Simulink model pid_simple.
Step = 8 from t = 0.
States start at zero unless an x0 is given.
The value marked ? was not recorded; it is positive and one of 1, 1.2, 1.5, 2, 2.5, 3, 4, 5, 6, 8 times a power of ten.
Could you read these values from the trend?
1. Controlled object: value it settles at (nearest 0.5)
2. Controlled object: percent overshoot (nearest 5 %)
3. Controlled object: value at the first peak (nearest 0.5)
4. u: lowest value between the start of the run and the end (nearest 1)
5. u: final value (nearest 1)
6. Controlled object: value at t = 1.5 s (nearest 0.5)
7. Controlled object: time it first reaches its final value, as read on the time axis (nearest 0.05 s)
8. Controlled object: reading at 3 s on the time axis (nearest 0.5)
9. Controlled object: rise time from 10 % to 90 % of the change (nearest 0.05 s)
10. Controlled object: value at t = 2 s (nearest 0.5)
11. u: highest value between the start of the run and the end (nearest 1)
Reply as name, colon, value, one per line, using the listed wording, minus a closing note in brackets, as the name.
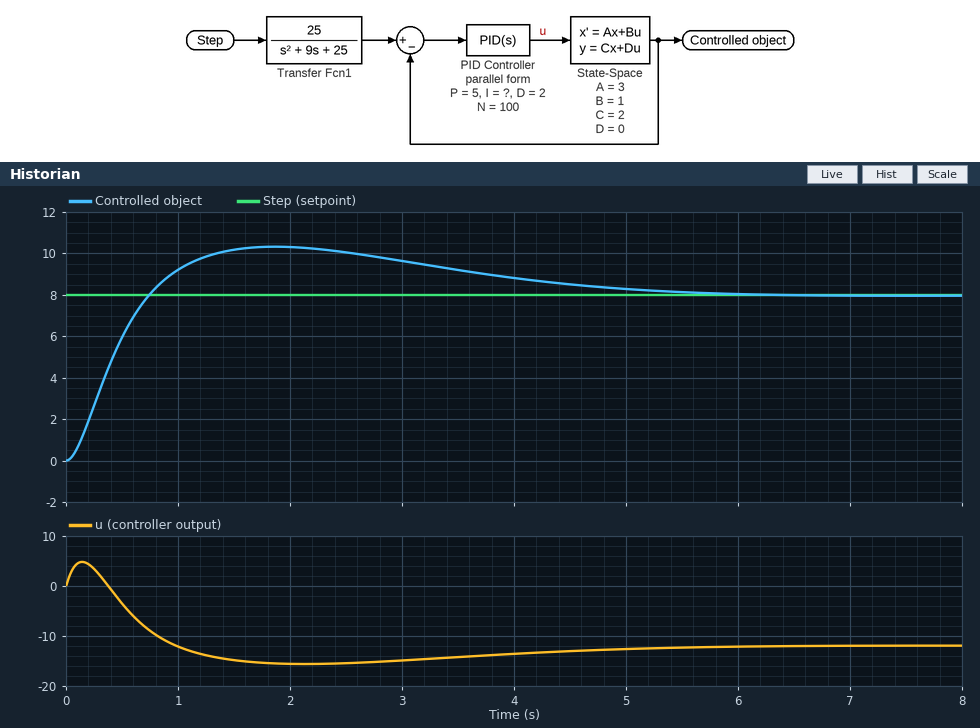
Controlled object: value it settles at: 8.0
Controlled object: percent overshoot: 30 %
Controlled object: value at the first peak: 10.5
u: lowest value between the start of the run and the end: -16
u: final value: -12
Controlled object: value at t = 1.5 s: 10.0
Controlled object: time it first reaches its final value, as read on the time axis: 0.75 s
Controlled object: reading at 3 s on the time axis: 9.5
Controlled object: rise time from 10 % to 90 % of the change: 0.50 s
Controlled object: value at t = 2 s: 10.5
u: highest value between the start of the run and the end: 5
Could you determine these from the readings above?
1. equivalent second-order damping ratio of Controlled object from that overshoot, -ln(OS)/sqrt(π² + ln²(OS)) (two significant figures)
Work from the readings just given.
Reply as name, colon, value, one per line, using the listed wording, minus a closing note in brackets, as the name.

equivalent second-order damping ratio of Controlled object from that overshoot, -ln(OS)/sqrt(π² + ln²(OS)): 0.36
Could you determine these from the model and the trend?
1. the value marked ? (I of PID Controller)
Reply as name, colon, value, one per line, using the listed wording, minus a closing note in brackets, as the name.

the value marked ?: 2
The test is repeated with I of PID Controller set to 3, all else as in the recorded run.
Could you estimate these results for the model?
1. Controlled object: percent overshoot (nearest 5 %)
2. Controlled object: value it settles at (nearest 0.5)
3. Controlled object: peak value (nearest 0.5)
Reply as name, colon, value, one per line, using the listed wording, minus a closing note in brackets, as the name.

Controlled object: percent overshoot: 25 %
Controlled object: value it settles at: 8.0
Controlled object: peak value: 10.0
